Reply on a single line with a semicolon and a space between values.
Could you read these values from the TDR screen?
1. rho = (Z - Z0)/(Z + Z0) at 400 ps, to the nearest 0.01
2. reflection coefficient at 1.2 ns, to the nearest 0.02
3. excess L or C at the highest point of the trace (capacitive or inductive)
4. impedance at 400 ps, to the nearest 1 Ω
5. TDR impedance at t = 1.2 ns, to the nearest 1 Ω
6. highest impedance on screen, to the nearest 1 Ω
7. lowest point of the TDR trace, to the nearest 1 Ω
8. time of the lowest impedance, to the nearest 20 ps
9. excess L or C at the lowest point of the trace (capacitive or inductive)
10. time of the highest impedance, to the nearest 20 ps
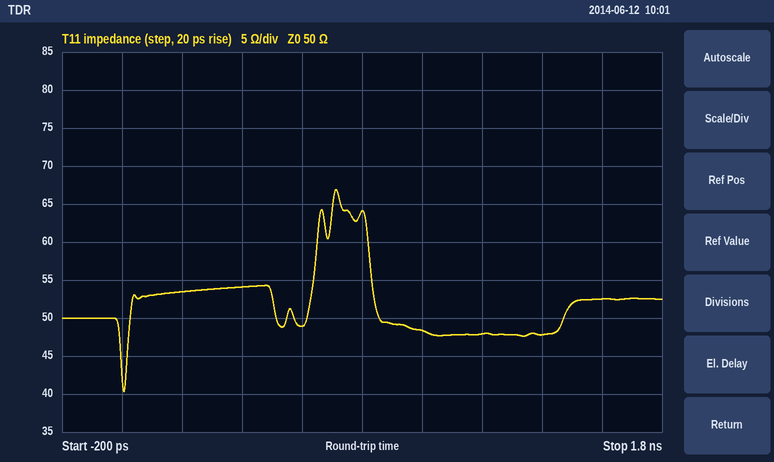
+0.04; -0.02; inductive; 54 Ω; 48 Ω; 67 Ω; 40 Ω; 0 ps; capacitive; 720 ps
